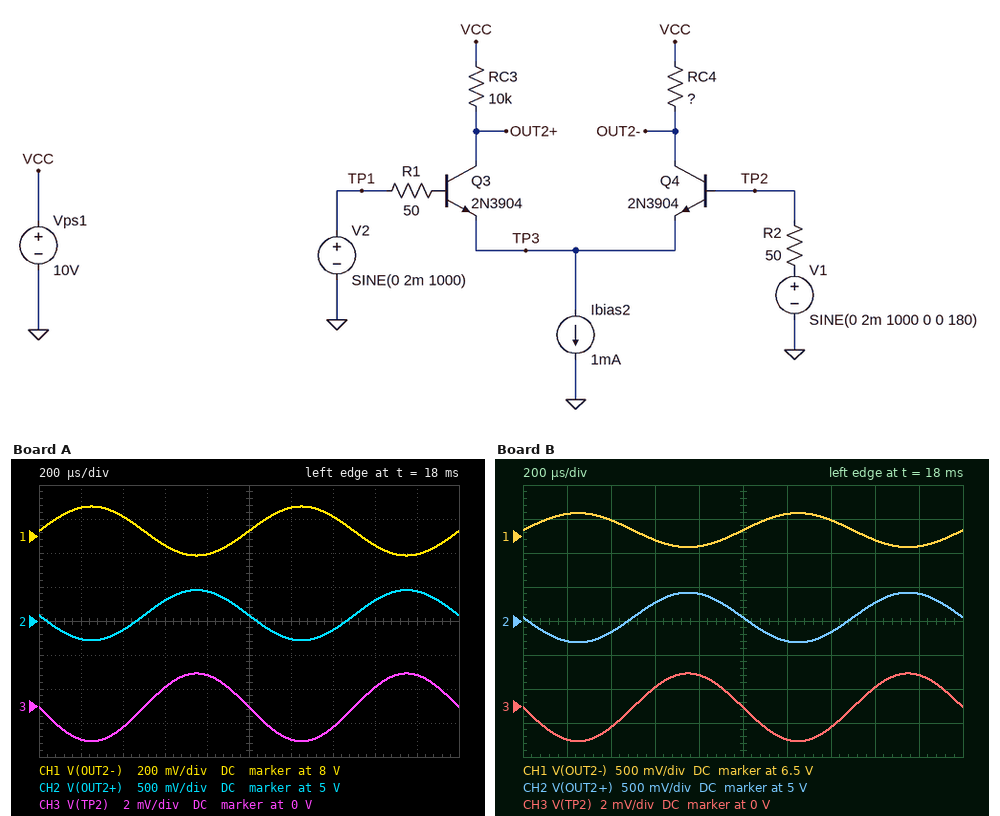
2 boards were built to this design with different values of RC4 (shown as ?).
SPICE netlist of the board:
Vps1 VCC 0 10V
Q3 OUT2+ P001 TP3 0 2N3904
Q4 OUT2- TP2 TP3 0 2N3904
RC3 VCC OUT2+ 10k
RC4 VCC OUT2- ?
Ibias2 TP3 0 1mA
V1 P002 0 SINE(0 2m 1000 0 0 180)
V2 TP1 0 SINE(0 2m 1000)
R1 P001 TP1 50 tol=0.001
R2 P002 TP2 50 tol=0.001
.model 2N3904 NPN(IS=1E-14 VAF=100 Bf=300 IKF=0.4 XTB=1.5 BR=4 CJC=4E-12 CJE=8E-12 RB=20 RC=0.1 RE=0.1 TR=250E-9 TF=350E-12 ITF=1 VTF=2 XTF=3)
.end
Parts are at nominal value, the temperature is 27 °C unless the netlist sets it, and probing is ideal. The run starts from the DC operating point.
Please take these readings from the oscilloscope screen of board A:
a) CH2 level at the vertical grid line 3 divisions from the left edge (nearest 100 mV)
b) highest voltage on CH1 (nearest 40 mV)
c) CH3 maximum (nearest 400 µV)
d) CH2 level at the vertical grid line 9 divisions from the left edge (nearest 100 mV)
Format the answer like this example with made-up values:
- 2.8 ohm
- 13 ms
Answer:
- 5.3 V
- 8.16 V
- 2.0 mV
- 5.4 V
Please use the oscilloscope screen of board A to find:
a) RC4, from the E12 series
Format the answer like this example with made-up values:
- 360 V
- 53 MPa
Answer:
- 3.9 kΩ
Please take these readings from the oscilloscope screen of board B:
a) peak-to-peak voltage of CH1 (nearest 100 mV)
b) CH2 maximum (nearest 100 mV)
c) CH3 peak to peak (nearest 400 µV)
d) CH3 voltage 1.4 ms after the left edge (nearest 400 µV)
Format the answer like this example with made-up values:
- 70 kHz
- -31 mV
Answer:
- 500 mV
- 5.4 V
- 4.0 mV
- -1.2 mV
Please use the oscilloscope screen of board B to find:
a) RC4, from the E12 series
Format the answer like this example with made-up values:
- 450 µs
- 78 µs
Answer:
- 6.8 kΩ
